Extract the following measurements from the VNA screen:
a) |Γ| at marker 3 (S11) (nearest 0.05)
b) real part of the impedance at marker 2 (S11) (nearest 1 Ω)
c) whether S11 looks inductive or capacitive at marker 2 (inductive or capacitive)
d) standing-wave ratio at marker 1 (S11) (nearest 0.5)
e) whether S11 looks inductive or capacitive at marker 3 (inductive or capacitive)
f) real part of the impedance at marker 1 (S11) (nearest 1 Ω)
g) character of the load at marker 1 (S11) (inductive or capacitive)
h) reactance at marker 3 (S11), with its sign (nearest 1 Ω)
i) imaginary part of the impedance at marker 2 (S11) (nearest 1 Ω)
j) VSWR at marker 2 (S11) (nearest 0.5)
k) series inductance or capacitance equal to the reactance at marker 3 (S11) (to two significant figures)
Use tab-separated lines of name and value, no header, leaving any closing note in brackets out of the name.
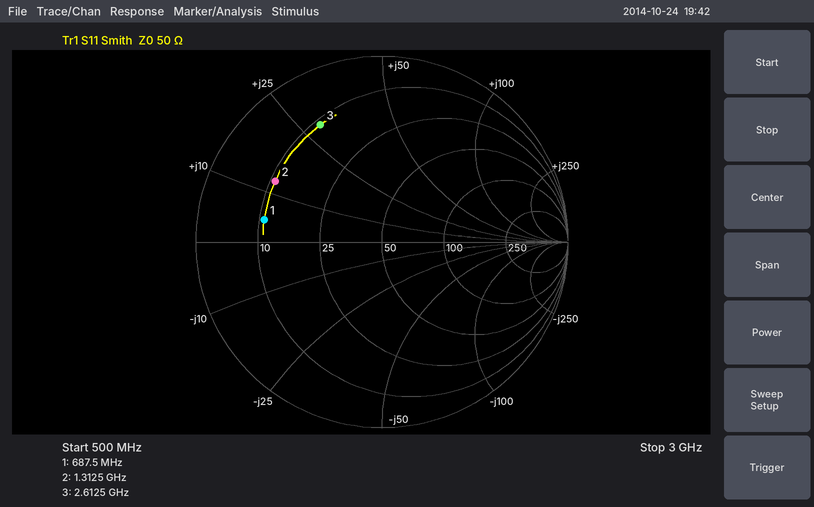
|Γ| at marker 3 (S11)	0.70
real part of the impedance at marker 2 (S11)	11 Ω
whether S11 looks inductive or capacitive at marker 2	inductive
standing-wave ratio at marker 1 (S11)	4.5
whether S11 looks inductive or capacitive at marker 3	inductive
real part of the impedance at marker 1 (S11)	11 Ω
character of the load at marker 1 (S11)	inductive
reactance at marker 3 (S11), with its sign	+29 Ω
imaginary part of the impedance at marker 2 (S11)	+13 Ω
VSWR at marker 2 (S11)	5.0
series inductance or capacitance equal to the reactance at marker 3 (S11)	1.8 nH
